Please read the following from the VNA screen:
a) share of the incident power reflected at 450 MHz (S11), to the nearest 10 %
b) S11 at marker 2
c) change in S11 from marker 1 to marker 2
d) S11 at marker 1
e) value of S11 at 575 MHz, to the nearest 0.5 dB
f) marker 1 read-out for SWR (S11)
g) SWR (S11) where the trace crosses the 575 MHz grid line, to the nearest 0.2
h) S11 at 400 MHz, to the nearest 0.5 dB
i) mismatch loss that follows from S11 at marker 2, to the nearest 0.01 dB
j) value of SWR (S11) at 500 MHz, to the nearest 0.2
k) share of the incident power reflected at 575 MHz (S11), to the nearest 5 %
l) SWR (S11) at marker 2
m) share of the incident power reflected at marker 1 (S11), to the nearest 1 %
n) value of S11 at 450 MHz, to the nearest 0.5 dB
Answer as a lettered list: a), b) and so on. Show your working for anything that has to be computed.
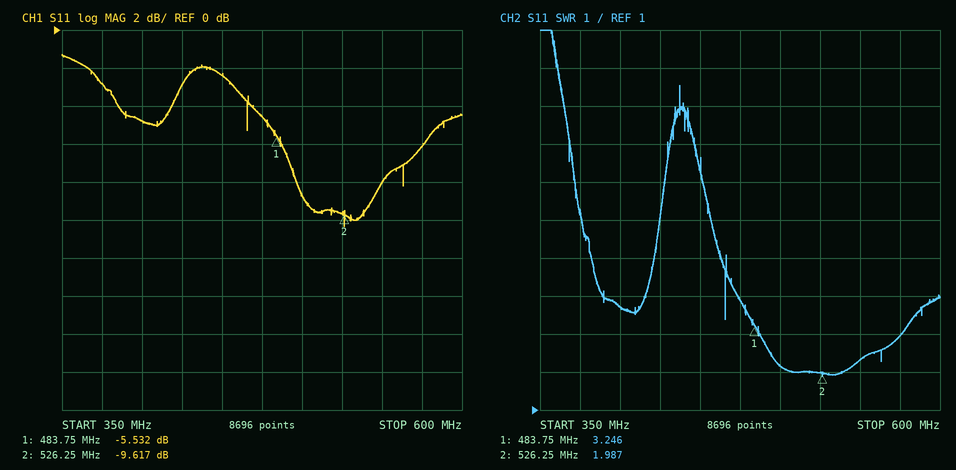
a) 10^(-2.5/10) ≈ 56.2 %, so 60 % to the nearest 10 %
b) -9.617 dB
c) -9.617 − (-5.532) = -4.085 dB
d) -5.532 dB
e) -6.0 dB
f) 3.246
g) 3.0
h) -5.0 dB
i) −10 log10(1 − 10^(-9.617/10)) ≈ 0.50 dB
j) 2.2
k) 10^(-6/10) ≈ 25 %
l) 1.987
m) 10^(-5.532/10) ≈ 28 %
n) -2.5 dB
